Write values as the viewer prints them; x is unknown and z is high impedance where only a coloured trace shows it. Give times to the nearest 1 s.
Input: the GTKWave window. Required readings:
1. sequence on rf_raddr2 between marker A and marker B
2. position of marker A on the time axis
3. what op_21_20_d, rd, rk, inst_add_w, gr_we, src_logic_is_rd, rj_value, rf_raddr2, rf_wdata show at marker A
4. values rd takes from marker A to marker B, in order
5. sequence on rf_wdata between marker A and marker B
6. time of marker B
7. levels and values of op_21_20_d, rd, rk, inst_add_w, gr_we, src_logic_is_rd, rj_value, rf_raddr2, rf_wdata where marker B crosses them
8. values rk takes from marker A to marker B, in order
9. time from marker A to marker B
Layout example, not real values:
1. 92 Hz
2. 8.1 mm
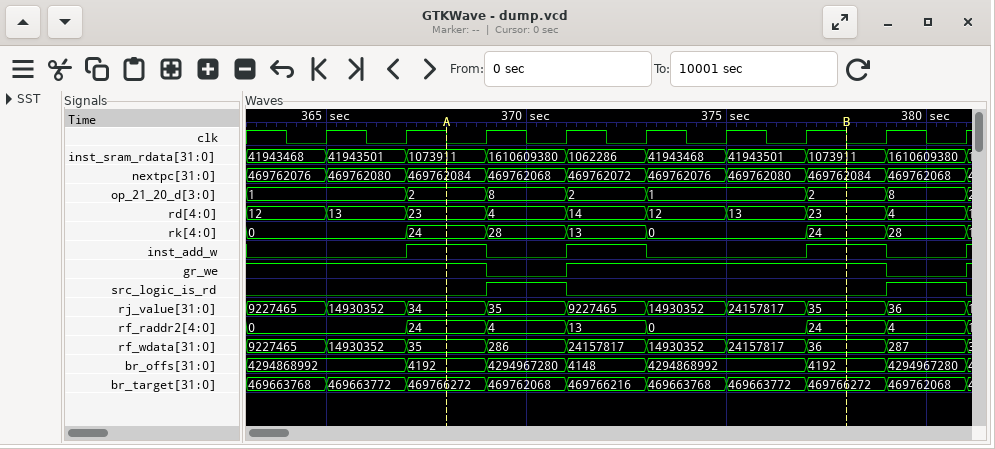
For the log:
1. 24, 4, 13, 0, 24
2. 368 s
3. op_21_20_d=2, rd=23, rk=24, inst_add_w=1, gr_we=1, src_logic_is_rd=0, rj_value=34, rf_raddr2=24, rf_wdata=35
4. 23, 4, 14, 12, 13, 23
5. 35, 286, 24157817, 14930352, 24157817, 36
6. 378 s
7. op_21_20_d=2, rd=23, rk=24, inst_add_w=1, gr_we=1, src_logic_is_rd=0, rj_value=35, rf_raddr2=24, rf_wdata=36
8. 24, 28, 13, 0, 24
9. 10 s
